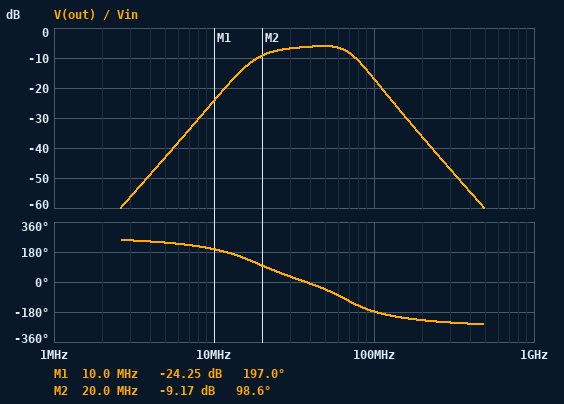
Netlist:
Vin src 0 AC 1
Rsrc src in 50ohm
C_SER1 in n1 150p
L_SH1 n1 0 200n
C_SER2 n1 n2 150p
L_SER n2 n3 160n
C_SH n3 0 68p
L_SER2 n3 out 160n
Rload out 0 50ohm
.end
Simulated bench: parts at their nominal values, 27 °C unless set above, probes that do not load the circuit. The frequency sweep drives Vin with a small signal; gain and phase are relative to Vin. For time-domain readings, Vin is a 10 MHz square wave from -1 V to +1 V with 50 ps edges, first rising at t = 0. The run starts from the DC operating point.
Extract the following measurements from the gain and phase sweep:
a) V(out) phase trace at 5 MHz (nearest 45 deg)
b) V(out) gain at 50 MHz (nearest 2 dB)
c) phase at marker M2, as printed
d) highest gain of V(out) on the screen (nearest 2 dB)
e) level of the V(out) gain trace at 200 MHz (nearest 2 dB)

225 deg
-6 dB
98.6 deg
-6 dB
-36 dB
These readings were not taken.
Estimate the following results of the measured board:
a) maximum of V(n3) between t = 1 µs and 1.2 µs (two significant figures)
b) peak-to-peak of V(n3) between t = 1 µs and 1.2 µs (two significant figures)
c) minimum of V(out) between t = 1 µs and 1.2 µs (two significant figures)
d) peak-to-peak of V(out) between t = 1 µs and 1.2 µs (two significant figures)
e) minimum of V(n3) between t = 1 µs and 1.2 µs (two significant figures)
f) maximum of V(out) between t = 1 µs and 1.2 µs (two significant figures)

530 mV
1.1 V
-360 mV
720 mV
-530 mV
360 mV
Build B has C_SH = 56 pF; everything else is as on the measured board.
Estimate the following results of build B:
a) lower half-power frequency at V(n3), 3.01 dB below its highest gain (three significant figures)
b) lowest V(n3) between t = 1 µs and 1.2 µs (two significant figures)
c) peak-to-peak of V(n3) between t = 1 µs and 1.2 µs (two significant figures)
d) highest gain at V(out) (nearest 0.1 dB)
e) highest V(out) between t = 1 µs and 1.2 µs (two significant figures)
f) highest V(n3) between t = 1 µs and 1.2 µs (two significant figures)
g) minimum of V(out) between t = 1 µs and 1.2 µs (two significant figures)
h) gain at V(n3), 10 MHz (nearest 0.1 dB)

35.3 MHz
-590 mV
1.2 V
-6.0 dB
390 mV
590 mV
-390 mV
-23.9 dB
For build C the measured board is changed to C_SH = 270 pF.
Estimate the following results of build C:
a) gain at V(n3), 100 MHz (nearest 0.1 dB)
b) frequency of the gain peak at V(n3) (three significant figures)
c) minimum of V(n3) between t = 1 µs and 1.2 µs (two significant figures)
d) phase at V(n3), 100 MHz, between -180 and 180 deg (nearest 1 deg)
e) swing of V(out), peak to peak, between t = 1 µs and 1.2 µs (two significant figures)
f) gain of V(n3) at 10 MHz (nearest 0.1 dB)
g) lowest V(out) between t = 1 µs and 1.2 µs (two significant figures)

-24.7 dB
25.3 MHz
-240 mV
-127 deg
430 mV
-26.9 dB
-210 mV
